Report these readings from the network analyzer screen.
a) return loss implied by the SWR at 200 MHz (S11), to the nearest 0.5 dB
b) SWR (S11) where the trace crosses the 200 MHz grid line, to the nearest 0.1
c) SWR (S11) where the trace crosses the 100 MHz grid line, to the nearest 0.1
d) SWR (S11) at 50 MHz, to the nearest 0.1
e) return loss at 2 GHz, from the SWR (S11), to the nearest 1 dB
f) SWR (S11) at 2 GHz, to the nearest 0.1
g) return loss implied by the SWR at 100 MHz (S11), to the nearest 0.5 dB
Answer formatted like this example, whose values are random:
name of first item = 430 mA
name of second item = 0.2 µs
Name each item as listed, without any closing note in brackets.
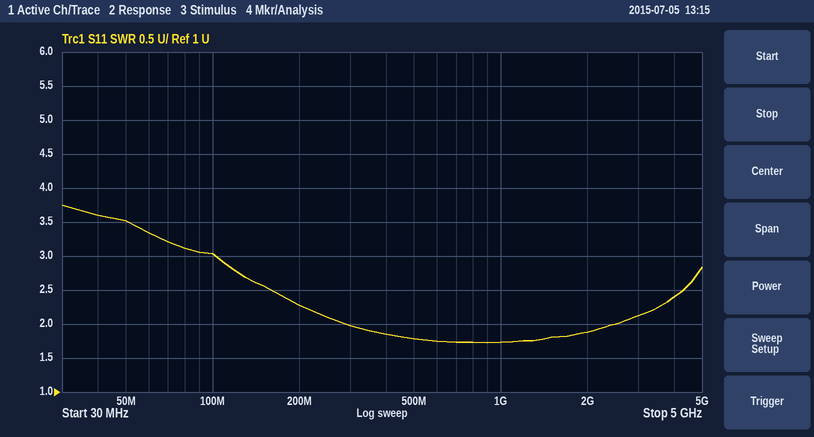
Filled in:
return loss implied by the SWR at 200 MHz (S11), to the nearest 0.5 dB = 8.0 dB
SWR (S11) where the trace crosses the 200 MHz grid line, to the nearest 0.1 = 2.3
SWR (S11) where the trace crosses the 100 MHz grid line, to the nearest 0.1 = 3.0
SWR (S11) at 50 MHz, to the nearest 0.1 = 3.5
return loss at 2 GHz, from the SWR (S11), to the nearest 1 dB = 10 dB
SWR (S11) at 2 GHz, to the nearest 0.1 = 1.9
return loss implied by the SWR at 100 MHz (S11), to the nearest 0.5 dB = 6.0 dB
